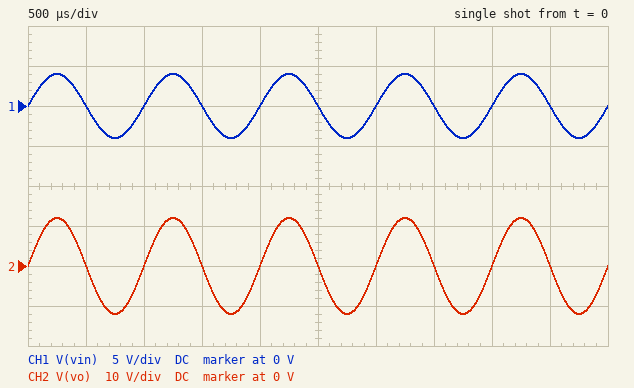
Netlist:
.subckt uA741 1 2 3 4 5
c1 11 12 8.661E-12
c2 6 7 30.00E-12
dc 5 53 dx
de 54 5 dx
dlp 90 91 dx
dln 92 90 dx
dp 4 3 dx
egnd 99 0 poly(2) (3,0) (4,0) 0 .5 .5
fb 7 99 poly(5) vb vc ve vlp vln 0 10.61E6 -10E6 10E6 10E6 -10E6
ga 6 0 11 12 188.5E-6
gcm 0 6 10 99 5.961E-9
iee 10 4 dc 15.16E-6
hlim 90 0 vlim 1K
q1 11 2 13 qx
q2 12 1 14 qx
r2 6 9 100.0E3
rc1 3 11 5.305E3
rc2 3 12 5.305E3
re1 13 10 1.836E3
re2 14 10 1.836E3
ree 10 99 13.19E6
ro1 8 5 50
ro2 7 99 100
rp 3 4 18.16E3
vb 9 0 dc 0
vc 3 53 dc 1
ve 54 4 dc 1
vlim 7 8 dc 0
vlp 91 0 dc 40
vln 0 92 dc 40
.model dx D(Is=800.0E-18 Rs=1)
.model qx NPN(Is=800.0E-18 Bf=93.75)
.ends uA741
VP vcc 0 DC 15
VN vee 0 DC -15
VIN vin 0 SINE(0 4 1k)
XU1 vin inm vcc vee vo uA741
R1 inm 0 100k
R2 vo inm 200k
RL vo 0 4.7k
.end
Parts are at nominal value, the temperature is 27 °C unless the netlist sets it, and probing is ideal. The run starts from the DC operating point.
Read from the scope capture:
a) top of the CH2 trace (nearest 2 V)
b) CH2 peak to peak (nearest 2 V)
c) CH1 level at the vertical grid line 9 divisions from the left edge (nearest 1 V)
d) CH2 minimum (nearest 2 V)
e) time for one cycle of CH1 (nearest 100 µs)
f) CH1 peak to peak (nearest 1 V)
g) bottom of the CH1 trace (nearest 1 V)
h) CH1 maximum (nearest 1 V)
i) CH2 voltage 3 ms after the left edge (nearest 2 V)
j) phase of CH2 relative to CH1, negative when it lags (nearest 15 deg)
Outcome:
12 V
24 V
0 V
-12 V
1.0 ms
8 V
-4 V
4 V
0 V
0 deg
